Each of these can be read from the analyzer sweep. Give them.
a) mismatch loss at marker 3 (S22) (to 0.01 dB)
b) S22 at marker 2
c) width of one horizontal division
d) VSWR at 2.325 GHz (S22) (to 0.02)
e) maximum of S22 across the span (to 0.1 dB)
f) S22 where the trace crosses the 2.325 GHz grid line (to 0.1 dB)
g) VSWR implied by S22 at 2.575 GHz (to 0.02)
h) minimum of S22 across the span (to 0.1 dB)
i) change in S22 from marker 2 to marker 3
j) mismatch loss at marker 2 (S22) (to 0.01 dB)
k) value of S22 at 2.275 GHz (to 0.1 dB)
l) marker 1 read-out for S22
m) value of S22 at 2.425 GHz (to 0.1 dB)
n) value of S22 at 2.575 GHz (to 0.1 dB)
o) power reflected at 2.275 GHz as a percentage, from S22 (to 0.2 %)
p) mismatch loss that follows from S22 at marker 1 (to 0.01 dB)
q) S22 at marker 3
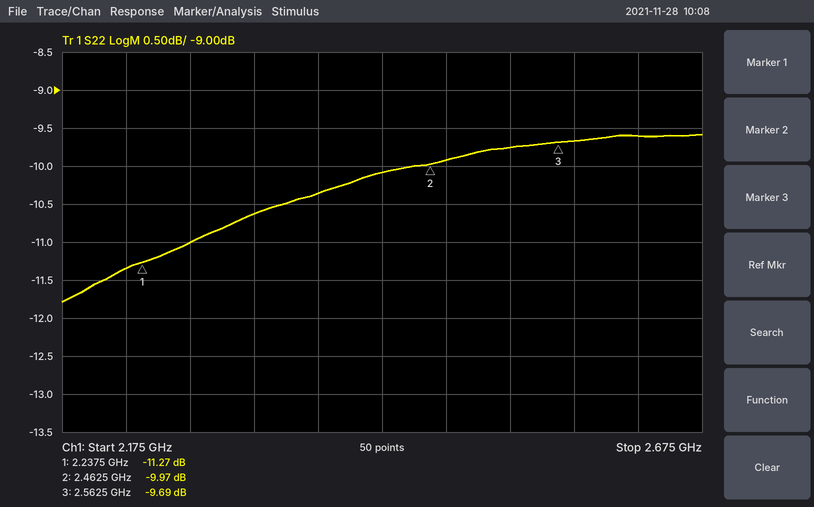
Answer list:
0.49 dB
-9.97 dB
50 MHz
1.84
-9.6 dB
-10.6 dB
1.98
-11.8 dB
0.28 dB
0.46 dB
-11.0 dB
-11.27 dB
-10.1 dB
-9.7 dB
8.0 %
0.34 dB
-9.69 dB
